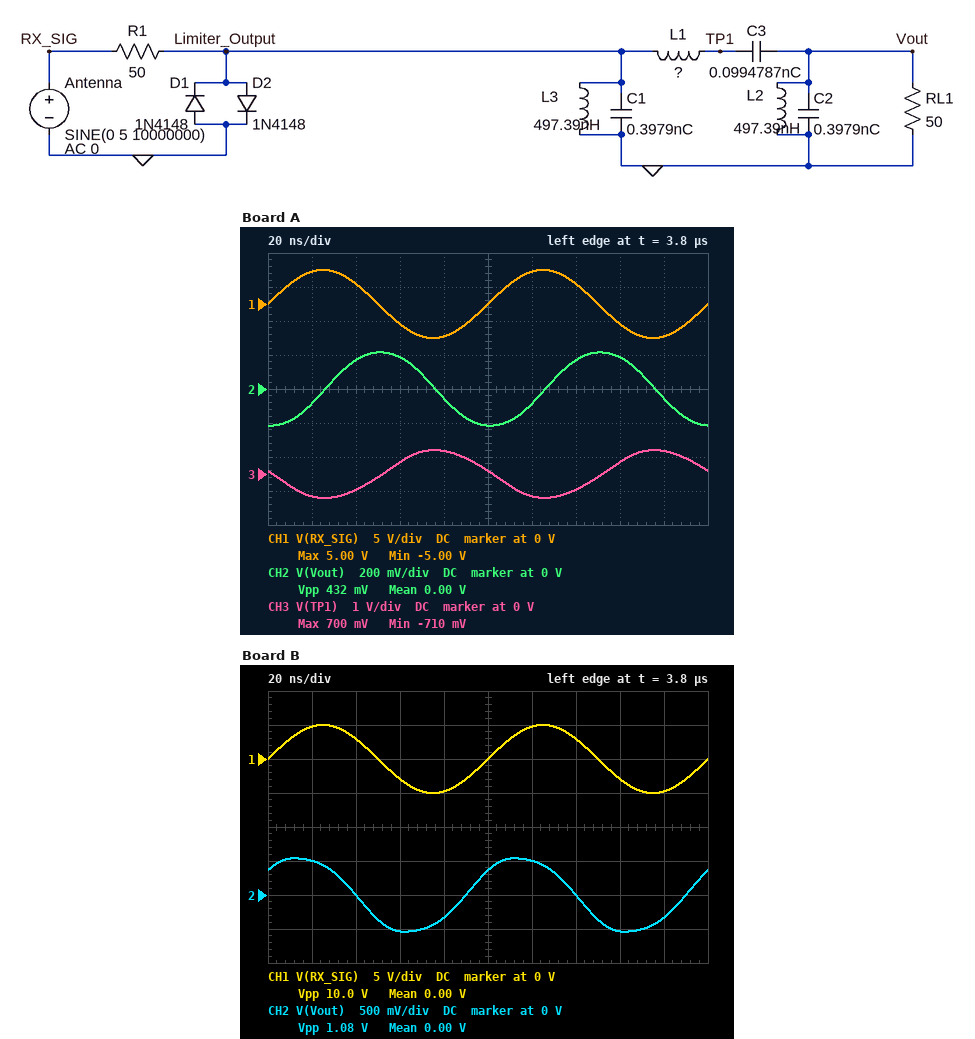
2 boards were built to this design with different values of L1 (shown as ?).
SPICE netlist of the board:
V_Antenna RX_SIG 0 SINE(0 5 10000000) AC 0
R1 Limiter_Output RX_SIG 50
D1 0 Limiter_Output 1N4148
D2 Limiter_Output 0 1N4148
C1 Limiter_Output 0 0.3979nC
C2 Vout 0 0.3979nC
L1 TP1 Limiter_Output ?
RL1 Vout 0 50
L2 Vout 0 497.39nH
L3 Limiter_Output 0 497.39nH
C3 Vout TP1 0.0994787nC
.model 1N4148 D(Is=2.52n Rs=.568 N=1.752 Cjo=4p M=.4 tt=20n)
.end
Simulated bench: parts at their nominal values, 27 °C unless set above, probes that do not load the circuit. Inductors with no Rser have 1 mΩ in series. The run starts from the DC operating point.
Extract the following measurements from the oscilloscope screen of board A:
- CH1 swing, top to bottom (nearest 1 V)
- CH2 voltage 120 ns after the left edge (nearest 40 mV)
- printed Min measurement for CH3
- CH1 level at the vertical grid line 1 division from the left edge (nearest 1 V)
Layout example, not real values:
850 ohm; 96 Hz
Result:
10 V; -80 mV; -710 mV; 5 V
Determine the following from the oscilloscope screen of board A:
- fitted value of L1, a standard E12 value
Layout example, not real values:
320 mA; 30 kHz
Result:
5.6 µH
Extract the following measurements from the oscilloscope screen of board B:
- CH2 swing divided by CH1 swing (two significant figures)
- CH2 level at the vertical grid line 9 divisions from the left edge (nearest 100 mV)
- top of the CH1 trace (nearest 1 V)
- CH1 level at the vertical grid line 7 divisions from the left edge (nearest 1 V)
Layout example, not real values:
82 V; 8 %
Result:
0.11; -300 mV; 5 V; 3 V
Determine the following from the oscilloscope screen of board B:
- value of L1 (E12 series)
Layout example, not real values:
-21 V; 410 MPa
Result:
1.2 µH
